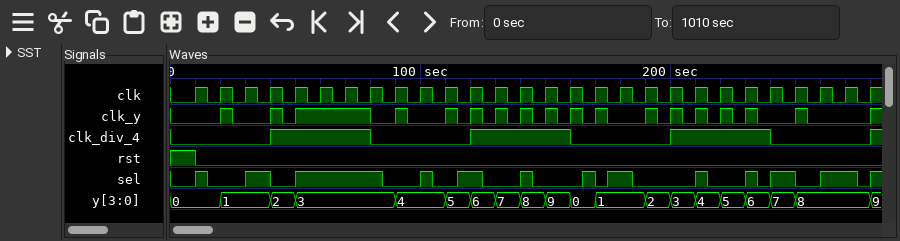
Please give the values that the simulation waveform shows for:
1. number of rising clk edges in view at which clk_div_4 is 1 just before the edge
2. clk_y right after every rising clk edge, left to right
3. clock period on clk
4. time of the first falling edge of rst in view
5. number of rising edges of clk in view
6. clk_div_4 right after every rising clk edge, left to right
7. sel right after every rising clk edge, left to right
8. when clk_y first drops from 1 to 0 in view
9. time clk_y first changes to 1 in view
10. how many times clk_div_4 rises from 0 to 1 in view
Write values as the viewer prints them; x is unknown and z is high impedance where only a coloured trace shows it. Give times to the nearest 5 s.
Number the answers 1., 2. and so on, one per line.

1. 12
2. 0 1 0 1 1 1 1 0 1 0 1 1 1 1 1 1 1 0 1 1 1 1 1 0 1 0 0 1
3. 10 s
4. 10 s
5. 28
6. 0 0 0 1 1 1 1 0 0 0 0 1 1 1 1 0 0 0 0 1 1 1 1 0 0 0 0 1
7. 1 0 1 0 1 1 1 1 0 1 0 1 0 1 0 0 0 1 0 0 1 0 1 1 0 1 1 1
8. 25 s
9. 20 s
10. 4
